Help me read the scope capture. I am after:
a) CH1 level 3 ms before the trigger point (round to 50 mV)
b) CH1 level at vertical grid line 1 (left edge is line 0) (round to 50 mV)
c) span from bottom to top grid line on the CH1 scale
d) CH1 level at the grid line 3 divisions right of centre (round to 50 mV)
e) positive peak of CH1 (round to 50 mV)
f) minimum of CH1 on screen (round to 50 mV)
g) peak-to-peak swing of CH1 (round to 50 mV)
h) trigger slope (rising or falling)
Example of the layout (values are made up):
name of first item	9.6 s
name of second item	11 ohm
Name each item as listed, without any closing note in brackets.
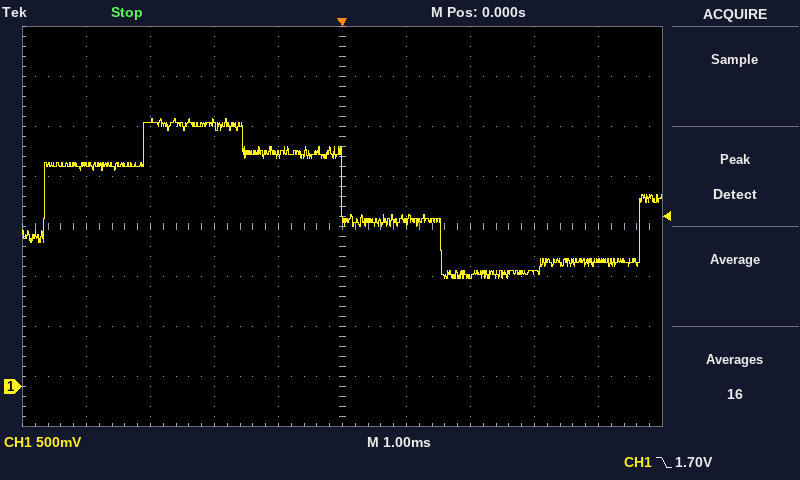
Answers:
CH1 level 3 ms before the trigger point	2.65 V
CH1 level at vertical grid line 1 (left edge is line 0)	2.20 V
span from bottom to top grid line on the CH1 scale	4 V
CH1 level at the grid line 3 divisions right of centre	1.15 V
positive peak of CH1	2.70 V
minimum of CH1 on screen	1.10 V
peak-to-peak swing of CH1	1.60 V
trigger slope	falling
